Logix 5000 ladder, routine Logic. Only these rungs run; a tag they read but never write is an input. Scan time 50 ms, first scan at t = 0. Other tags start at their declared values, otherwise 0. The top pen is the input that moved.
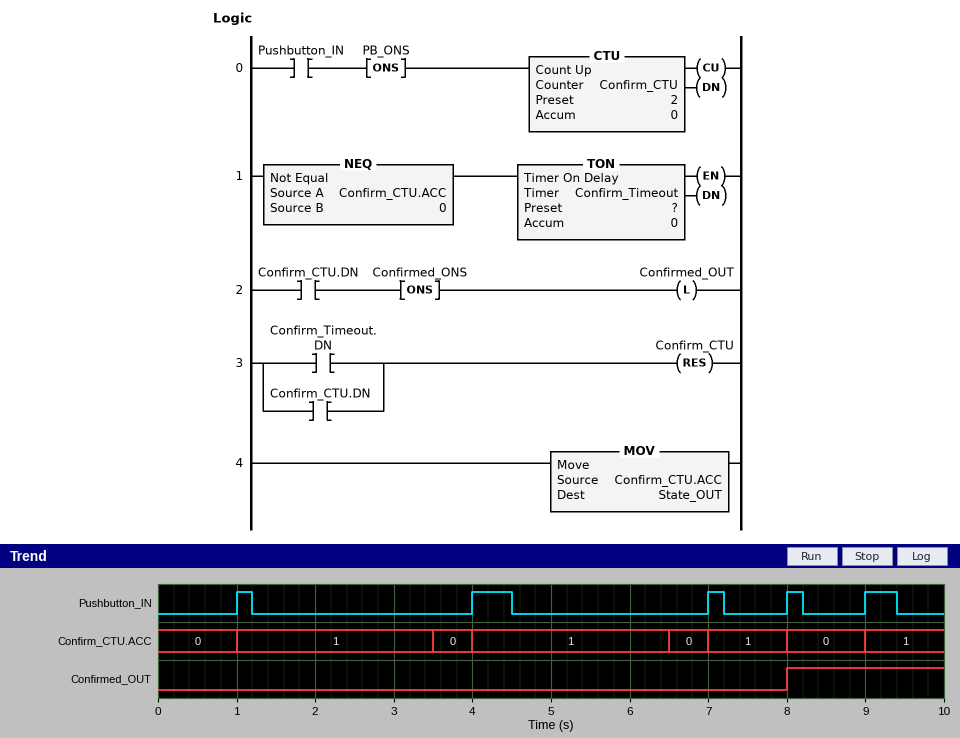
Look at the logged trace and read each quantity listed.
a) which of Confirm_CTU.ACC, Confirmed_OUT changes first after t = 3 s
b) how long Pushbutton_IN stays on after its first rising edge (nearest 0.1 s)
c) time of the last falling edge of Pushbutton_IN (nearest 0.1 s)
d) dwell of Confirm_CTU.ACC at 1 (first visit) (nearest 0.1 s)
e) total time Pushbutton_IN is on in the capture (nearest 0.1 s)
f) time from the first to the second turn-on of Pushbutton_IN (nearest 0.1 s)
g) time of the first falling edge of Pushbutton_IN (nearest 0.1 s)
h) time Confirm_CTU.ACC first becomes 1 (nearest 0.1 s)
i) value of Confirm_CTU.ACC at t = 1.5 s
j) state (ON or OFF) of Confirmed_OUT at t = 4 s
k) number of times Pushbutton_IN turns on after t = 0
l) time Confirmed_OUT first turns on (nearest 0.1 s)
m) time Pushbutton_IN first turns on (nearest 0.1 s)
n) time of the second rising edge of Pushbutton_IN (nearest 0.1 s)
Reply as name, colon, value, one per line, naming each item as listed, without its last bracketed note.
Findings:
which of Confirm_CTU.ACC, Confirmed_OUT changes first after t = 3 s: Confirm_CTU.ACC
how long Pushbutton_IN stays on after its first rising edge: 0.2 s
time of the last falling edge of Pushbutton_IN: 9.4 s
dwell of Confirm_CTU.ACC at 1 (first visit): 2.5 s
total time Pushbutton_IN is on in the capture: 1.5 s
time from the first to the second turn-on of Pushbutton_IN: 3.0 s
time of the first falling edge of Pushbutton_IN: 1.2 s
time Confirm_CTU.ACC first becomes 1: 1.0 s
value of Confirm_CTU.ACC at t = 1.5 s: 1
state (ON or OFF) of Confirmed_OUT at t = 4 s: OFF
number of times Pushbutton_IN turns on after t = 0: 5
time Confirmed_OUT first turns on: 8.0 s
time Pushbutton_IN first turns on: 1.0 s
time of the second rising edge of Pushbutton_IN: 4.0 s
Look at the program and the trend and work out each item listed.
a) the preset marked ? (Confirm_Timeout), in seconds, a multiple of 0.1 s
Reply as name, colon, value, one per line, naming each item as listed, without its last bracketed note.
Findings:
the preset marked ? (Confirm_Timeout), in seconds, a multiple of 0.1 s: 2.5 s
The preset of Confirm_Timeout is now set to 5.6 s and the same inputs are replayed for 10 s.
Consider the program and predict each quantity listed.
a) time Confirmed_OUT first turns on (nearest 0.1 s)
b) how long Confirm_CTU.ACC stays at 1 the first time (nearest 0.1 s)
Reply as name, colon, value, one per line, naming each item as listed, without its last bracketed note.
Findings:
time Confirmed_OUT first turns on: 4.0 s
how long Confirm_CTU.ACC stays at 1 the first time: 3.0 s
